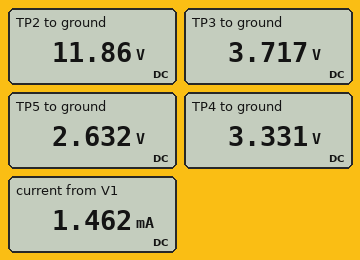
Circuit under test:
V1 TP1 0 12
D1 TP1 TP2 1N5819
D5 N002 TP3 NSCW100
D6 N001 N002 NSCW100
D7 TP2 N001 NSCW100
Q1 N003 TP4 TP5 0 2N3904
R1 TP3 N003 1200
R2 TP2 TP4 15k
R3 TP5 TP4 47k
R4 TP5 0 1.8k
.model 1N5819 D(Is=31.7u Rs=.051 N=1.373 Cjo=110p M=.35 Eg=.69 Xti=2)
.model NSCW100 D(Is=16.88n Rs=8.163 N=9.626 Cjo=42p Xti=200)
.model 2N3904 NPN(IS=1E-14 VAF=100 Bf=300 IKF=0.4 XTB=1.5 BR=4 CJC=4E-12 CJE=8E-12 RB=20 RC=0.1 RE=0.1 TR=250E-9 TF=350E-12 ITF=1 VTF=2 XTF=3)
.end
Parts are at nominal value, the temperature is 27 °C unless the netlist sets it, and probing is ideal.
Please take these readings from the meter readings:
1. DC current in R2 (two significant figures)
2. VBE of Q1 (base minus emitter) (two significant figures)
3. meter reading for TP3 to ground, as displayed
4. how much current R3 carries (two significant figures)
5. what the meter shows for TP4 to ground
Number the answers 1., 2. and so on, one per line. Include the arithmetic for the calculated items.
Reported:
1. (11.86 V - 3.331 V) / 15 kΩ = 570 µA
2. 3.331 V - 2.632 V = 700 mV
3. 3.717 V
4. (3.331 V - 2.632 V) / 47 kΩ = 15 µA
5. 3.331 V
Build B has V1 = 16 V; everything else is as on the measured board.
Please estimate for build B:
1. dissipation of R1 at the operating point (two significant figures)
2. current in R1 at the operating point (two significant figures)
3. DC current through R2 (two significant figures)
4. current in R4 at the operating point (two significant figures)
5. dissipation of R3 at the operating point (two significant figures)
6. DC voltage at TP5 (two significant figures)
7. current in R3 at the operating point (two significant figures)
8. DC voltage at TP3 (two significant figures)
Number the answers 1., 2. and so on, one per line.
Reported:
1. 4.5 mW
2. 1.9 mA
3. 690 µA
4. 2.6 mA
5. 11 µW
6. 4.7 V
7. 15 µA
8. 7.1 V
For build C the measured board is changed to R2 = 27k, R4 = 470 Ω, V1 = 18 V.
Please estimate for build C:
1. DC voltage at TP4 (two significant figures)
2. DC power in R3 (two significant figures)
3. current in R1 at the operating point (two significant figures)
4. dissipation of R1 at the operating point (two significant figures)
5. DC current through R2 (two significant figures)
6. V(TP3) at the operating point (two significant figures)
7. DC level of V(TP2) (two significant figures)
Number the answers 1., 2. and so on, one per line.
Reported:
1. 3.2 V
2. 11 µW
3. 4.8 mA
4. 28 mW
5. 540 µA
6. 8.3 V
7. 18 V
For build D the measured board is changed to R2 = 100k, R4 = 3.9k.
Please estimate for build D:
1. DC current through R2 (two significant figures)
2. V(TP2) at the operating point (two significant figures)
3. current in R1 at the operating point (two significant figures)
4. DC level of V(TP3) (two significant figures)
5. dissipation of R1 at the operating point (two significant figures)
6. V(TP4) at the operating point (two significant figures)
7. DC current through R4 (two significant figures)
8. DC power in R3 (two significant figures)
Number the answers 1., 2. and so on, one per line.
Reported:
1. 82 µA
2. 12 V
3. 700 µA
4. 3.9 V
5. 590 µW
6. 3.7 V
7. 780 µA
8. 9.2 µW
